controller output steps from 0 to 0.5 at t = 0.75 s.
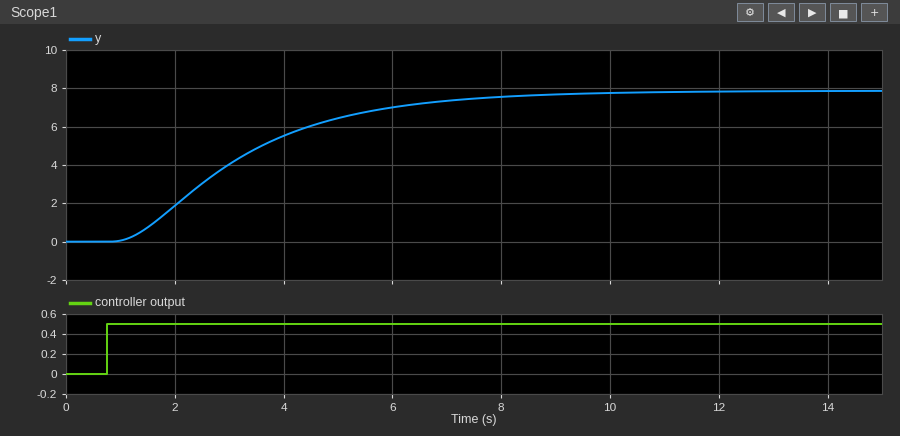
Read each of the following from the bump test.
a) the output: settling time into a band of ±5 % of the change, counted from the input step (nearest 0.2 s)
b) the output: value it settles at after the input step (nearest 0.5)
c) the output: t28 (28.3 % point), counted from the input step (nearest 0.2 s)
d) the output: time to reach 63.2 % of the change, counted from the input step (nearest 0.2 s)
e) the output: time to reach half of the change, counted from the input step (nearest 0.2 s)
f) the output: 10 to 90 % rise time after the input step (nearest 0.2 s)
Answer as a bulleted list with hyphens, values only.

- 6.8 s
- 8.0
- 1.4 s
- 2.8 s
- 2.2 s
- 4.6 s
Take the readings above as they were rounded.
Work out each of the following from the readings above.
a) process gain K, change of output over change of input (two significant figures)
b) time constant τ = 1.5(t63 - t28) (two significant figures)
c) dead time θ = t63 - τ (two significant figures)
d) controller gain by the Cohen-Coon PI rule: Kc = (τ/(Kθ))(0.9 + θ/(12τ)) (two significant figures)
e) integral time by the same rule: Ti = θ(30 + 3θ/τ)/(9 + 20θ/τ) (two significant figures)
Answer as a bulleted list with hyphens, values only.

- 16
- 2.1 s
- 0.70 s
- 0.17
- 1.4 s
